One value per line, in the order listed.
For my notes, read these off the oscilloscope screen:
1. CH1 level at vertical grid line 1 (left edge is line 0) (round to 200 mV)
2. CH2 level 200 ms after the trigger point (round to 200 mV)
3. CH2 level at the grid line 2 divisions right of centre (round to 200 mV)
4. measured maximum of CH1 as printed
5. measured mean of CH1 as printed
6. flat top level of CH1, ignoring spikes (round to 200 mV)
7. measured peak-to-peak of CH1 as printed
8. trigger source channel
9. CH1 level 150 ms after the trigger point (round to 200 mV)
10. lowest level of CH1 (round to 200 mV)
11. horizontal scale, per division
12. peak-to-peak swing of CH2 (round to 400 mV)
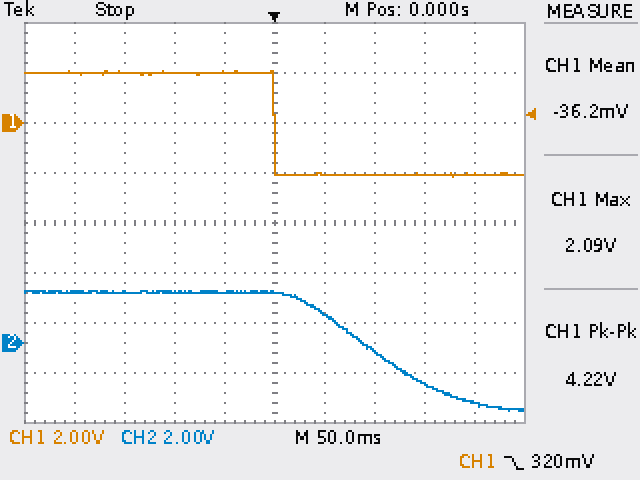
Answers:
2.0 V
-2.4 V
-400 mV
2.09 V
-36.2 mV
2.0 V
4.22 V
CH1
-2.0 V
-2.2 V
50 ms
4.8 V
